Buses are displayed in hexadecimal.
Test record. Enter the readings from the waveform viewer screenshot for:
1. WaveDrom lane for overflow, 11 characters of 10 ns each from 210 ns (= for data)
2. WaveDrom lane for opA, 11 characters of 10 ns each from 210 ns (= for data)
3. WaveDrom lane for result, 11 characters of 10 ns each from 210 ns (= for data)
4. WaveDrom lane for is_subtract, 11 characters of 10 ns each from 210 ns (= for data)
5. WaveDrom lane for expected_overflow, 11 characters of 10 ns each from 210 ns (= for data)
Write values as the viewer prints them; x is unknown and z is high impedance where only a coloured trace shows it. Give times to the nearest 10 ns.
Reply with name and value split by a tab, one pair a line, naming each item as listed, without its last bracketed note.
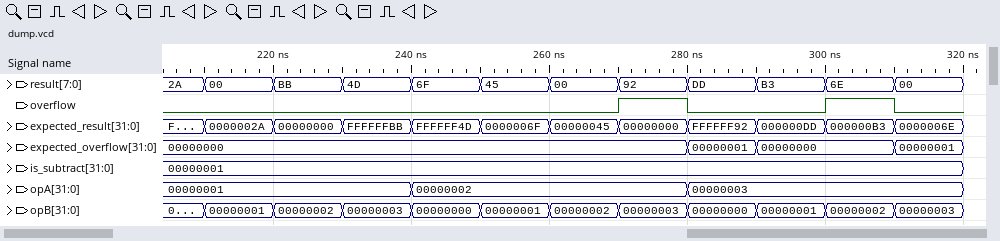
WaveDrom lane for overflow, 11 characters of 10 ns each from 210 ns	{name: 'overflow', wave: '0.....10.10'}
WaveDrom lane for opA, 11 characters of 10 ns each from 210 ns	{name: 'opA', wave: '=..=...=...', data: '00000001 00000002 00000003'}
WaveDrom lane for result, 11 characters of 10 ns each from 210 ns	{name: 'result', wave: '===========', data: '00 BB 4D 6F 45 00 92 DD B3 6E 00'}
WaveDrom lane for is_subtract, 11 characters of 10 ns each from 210 ns	{name: 'is_subtract', wave: '=..........', data: '00000001'}
WaveDrom lane for expected_overflow, 11 characters of 10 ns each from 210 ns	{name: 'expected_overflow', wave: '=......==.=', data: '00000000 00000001 00000000 00000001'}
